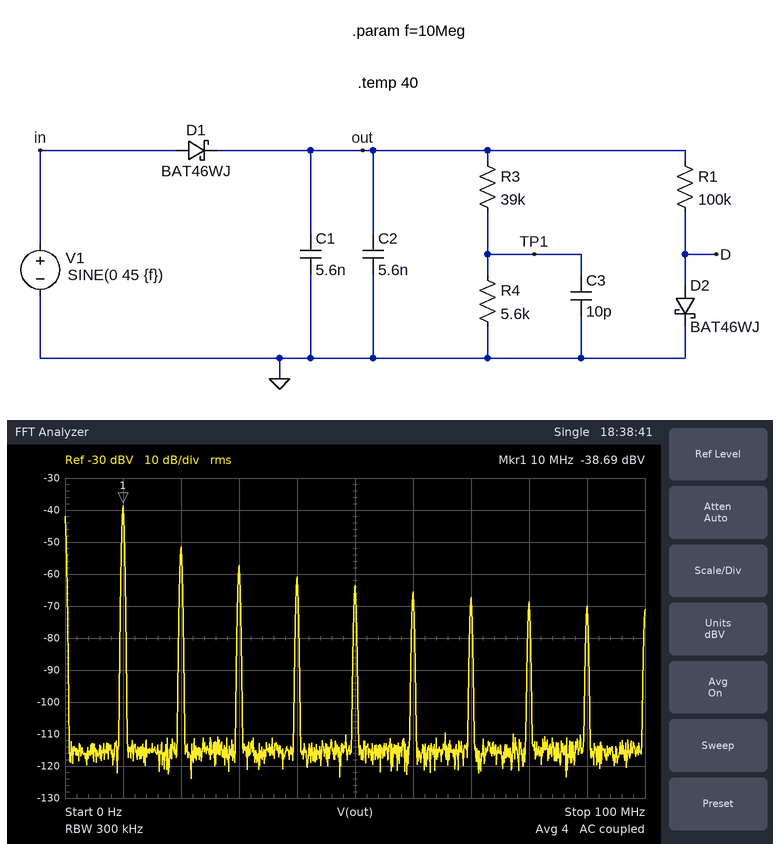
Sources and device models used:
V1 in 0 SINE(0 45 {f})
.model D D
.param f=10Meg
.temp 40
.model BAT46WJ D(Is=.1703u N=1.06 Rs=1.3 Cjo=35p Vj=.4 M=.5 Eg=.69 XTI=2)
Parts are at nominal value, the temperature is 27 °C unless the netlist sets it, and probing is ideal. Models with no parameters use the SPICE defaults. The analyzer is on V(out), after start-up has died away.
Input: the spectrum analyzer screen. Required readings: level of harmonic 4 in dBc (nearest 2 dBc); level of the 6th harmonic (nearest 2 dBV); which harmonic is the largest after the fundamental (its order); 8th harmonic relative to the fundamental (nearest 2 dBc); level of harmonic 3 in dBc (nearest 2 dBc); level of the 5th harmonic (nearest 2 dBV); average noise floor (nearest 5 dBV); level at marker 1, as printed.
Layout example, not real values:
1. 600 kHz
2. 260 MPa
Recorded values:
1. -22 dBc
2. -66 dBV
3. 2
4. -30 dBc
5. -18 dBc
6. -64 dBV
7. -115 dBV
8. -38.69 dBV
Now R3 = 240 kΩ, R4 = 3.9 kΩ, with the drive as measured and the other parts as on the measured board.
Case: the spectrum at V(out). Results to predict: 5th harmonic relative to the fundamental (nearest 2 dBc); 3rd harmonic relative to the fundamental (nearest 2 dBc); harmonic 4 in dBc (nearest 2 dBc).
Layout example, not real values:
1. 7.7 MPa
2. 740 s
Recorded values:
1. -28 dBc
2. -20 dBc
3. -26 dBc
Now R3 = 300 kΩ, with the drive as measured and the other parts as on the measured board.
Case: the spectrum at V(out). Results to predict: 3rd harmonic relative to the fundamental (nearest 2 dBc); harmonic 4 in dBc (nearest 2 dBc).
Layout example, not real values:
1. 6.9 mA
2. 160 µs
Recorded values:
1. -20 dBc
2. -26 dBc
